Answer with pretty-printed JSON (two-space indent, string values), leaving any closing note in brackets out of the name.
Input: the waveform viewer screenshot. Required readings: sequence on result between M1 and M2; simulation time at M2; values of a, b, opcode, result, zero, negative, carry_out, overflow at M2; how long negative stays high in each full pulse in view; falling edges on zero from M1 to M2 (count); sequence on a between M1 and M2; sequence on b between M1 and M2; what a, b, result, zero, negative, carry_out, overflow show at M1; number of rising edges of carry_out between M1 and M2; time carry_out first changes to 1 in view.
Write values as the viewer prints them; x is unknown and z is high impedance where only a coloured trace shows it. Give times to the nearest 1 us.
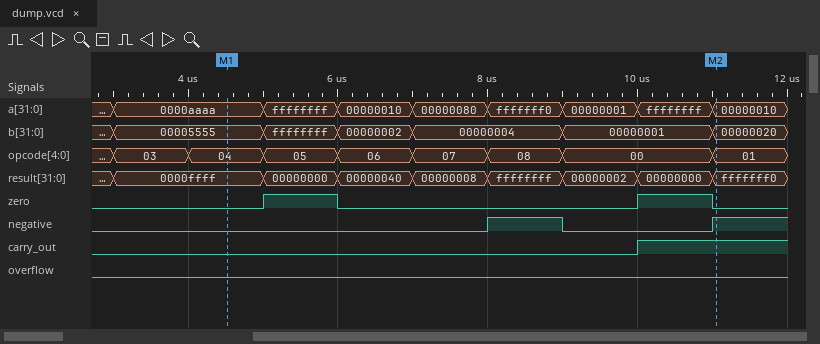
{
  "sequence on result between M1 and M2": "0000ffff, 00000000, 00000040, 00000008, ffffffff, 00000002, 00000000, fffffff0",
  "simulation time at M2": "11 us",
  "values of a, b, opcode, result, zero, negative, carry_out, overflow at M2": "a=00000010, b=00000020, opcode=01, result=fffffff0, zero=0, negative=1, carry_out=1, overflow=0",
  "how long negative stays high in each full pulse in view": "1 us",
  "falling edges on zero from M1 to M2": "2",
  "sequence on a between M1 and M2": "0000aaaa, ffffffff, 00000010, 00000080, fffffff0, 00000001, ffffffff, 00000010",
  "sequence on b between M1 and M2": "00005555, ffffffff, 00000002, 00000004, 00000001, 00000020",
  "what a, b, result, zero, negative, carry_out, overflow show at M1": "a=0000aaaa, b=00005555, result=0000ffff, zero=0, negative=0, carry_out=0, overflow=0",
  "number of rising edges of carry_out between M1 and M2": "1",
  "time carry_out first changes to 1 in view": "10 us"
}
